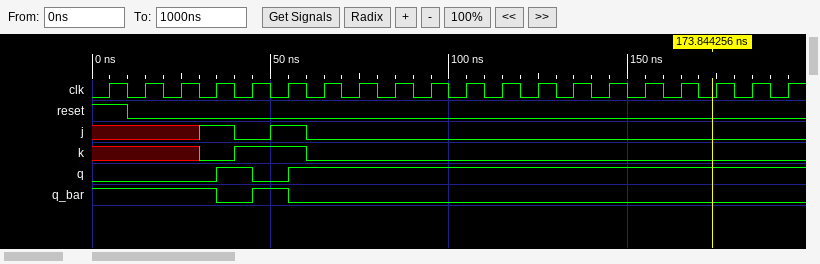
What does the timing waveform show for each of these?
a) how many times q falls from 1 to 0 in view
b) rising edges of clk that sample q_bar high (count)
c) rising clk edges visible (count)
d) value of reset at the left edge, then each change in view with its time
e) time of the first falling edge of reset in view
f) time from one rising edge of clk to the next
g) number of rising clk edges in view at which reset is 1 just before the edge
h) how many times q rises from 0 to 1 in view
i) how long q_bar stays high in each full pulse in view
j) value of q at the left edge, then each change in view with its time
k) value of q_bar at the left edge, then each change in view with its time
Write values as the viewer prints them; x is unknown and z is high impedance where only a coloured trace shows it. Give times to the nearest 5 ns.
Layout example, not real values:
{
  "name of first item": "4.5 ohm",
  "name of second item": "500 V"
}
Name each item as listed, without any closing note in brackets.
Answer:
{
  "how many times q falls from 1 to 0 in view": "1",
  "rising edges of clk that sample q_bar high": "5",
  "rising clk edges visible": "20",
  "value of reset at the left edge, then each change in view with its time": "1, 0 at 10 ns",
  "time of the first falling edge of reset in view": "10 ns",
  "time from one rising edge of clk to the next": "10 ns",
  "number of rising clk edges in view at which reset is 1 just before the edge": "1",
  "how many times q rises from 0 to 1 in view": "2",
  "how long q_bar stays high in each full pulse in view": "10 ns",
  "value of q at the left edge, then each change in view with its time": "0, 1 at 35 ns, 0 at 45 ns, 1 at 55 ns",
  "value of q_bar at the left edge, then each change in view with its time": "1, 0 at 35 ns, 1 at 45 ns, 0 at 55 ns"
}
